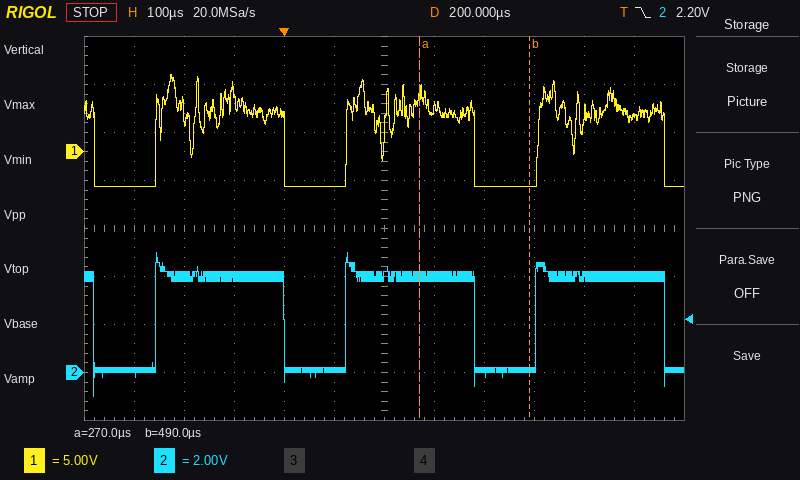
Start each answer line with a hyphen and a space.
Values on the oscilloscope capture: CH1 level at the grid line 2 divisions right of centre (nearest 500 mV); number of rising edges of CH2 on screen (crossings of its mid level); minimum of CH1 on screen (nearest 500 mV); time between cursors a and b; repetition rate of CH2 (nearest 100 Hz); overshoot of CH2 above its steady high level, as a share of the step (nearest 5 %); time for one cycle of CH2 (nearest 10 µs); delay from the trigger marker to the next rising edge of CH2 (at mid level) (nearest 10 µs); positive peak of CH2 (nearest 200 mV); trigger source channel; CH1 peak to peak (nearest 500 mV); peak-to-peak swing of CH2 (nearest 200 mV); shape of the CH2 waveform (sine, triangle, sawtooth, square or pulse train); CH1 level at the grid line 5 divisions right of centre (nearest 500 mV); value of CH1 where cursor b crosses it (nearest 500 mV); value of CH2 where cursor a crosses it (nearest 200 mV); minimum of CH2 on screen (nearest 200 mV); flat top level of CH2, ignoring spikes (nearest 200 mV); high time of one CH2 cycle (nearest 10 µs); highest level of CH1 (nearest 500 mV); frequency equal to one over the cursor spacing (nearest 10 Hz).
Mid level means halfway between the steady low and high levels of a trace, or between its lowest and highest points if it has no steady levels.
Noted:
- -3.5 V
- 3
- -3.5 V
- 220 µs
- 2.6 kHz
- 25 %
- 380 µs
- 120 µs
- 5.0 V
- CH2
- 11.5 V
- 6.0 V
- pulse train
- 3.5 V
- -3.5 V
- 4.0 V
- -1.0 V
- 4.0 V
- 260 µs
- 8.0 V
- 4.55 kHz
